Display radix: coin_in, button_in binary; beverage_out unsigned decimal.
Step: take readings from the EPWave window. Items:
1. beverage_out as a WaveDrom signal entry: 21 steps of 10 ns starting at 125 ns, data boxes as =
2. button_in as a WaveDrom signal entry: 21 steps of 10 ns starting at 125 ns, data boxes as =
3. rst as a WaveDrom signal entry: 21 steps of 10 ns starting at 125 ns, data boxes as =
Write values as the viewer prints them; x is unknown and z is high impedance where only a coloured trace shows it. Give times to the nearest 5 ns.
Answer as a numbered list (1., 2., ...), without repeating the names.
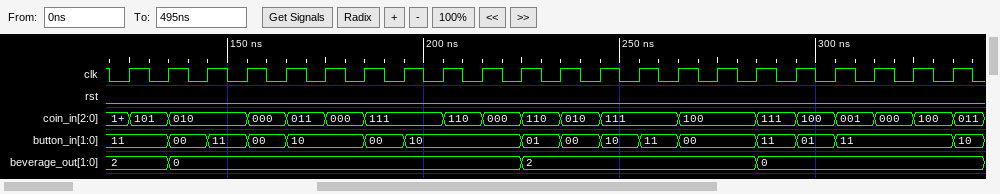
1. {name: 'beverage_out', wave: '==........=.....=....', data: '2 0 2 0'}
2. {name: 'button_in', wave: '=====.==..=====.===..', data: '11 00 11 00 10 00 10 01 00 10 11 00 11 01 11'}
3. {name: 'rst', wave: '0....................'}
